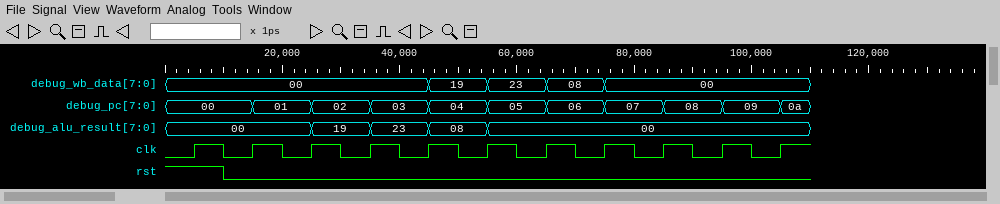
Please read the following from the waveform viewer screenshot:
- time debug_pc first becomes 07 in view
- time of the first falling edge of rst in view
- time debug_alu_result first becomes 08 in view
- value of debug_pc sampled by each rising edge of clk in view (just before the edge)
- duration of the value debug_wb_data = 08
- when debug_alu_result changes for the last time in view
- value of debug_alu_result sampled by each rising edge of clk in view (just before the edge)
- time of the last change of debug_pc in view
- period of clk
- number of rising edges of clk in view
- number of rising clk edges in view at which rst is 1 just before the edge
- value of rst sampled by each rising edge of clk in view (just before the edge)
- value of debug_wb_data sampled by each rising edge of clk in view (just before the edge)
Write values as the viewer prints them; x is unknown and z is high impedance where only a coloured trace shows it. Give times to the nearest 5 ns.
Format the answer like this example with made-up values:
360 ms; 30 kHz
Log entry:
75 ns; 10 ns; 45 ns; 00, 00, 01, 02, 03, 04, 05, 06, 07, 08, 09; 10 ns; 55 ns; 00, 00, 00, 19, 23, 08, 00, 00, 00, 00, 00; 105 ns; 10 ns; 11; 1; 1 0 0 0 0 0 0 0 0 0 0; 00, 00, 00, 00, 00, 19, 23, 08, 00, 00, 00
